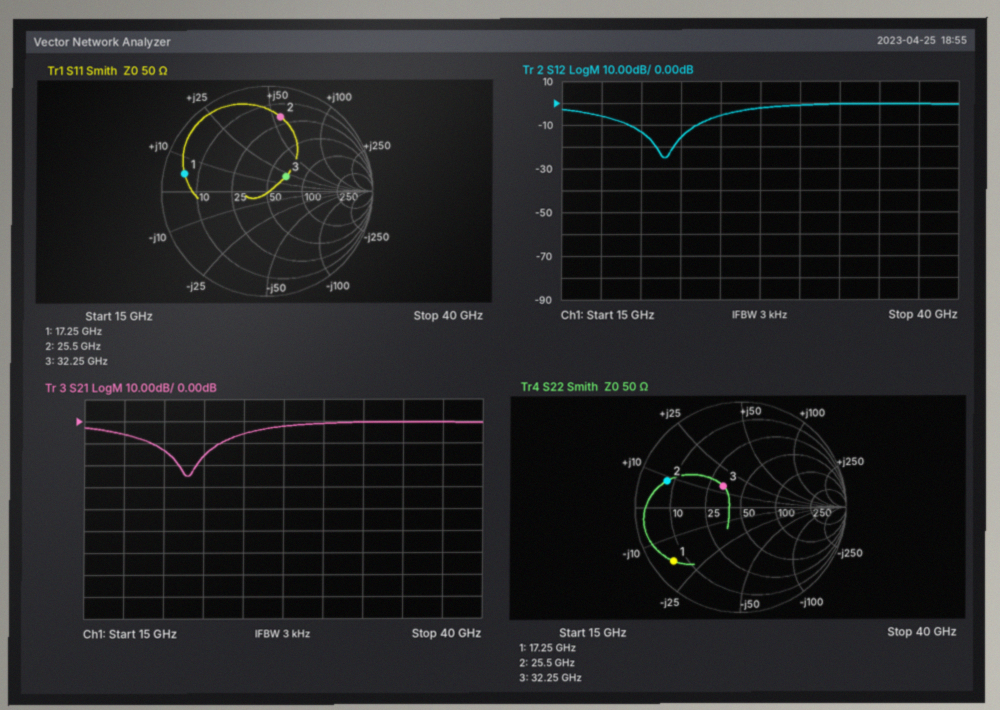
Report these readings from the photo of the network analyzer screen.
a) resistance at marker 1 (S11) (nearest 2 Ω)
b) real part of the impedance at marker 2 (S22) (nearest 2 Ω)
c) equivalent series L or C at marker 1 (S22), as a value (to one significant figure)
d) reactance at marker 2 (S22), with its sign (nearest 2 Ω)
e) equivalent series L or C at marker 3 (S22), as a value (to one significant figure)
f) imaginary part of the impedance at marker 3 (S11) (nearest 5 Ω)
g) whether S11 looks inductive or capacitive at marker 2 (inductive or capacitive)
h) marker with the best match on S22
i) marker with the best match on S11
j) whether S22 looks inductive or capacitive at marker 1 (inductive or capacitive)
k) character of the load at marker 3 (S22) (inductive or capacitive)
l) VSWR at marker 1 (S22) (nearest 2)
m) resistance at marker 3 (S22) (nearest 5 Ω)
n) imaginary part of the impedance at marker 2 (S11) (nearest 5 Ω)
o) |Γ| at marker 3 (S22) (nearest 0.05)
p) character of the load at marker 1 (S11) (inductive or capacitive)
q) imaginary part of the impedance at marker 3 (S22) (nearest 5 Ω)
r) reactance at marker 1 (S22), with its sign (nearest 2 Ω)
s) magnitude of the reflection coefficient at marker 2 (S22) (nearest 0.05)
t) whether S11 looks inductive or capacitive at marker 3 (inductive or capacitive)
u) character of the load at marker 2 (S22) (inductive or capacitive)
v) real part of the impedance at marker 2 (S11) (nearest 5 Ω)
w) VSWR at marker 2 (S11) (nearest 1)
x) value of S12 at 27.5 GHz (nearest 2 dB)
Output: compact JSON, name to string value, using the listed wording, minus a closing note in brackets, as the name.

{"resistance at marker 1 (S11)": "6 Ω", "real part of the impedance at marker 2 (S22)": "8 Ω", "equivalent series L or C at marker 1 (S22), as a value": "500 fF", "reactance at marker 2 (S22), with its sign": "+8 Ω", "equivalent series L or C at marker 3 (S22), as a value": "70 pH", "imaginary part of the impedance at marker 3 (S11)": "+20 Ω", "whether S11 looks inductive or capacitive at marker 2": "inductive", "marker with the best match on S22": "marker 3", "marker with the best match on S11": "marker 3", "whether S22 looks inductive or capacitive at marker 1": "capacitive", "character of the load at marker 3 (S22)": "inductive", "VSWR at marker 1 (S22)": "10", "resistance at marker 3 (S22)": "35 Ω", "imaginary part of the impedance at marker 2 (S11)": "+55 Ω", "|Γ| at marker 3 (S22)": "0.25", "character of the load at marker 1 (S11)": "inductive", "imaginary part of the impedance at marker 3 (S22)": "+15 Ω", "reactance at marker 1 (S22), with its sign": "-18 Ω", "magnitude of the reflection coefficient at marker 2 (S22)": "0.75", "whether S11 looks inductive or capacitive at marker 3": "inductive", "character of the load at marker 2 (S22)": "inductive", "real part of the impedance at marker 2 (S11)": "20 Ω", "VSWR at marker 2 (S11)": "6", "value of S12 at 27.5 GHz": "-2 dB"}
